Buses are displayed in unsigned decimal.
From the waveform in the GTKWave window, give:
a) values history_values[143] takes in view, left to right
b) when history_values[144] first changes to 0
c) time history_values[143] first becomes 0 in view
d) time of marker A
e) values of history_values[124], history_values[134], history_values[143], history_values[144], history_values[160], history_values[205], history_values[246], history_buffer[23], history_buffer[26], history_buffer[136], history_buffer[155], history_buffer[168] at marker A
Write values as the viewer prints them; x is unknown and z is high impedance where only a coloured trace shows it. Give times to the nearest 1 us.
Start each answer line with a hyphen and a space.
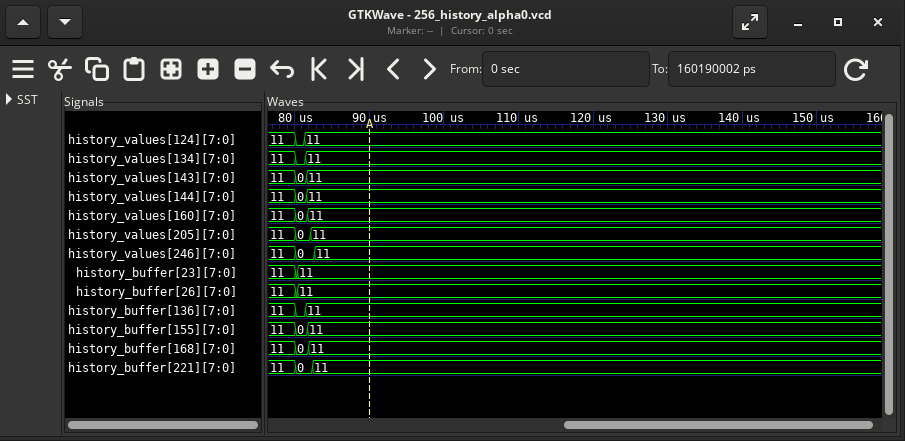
- 11, 0, 11
- 80 us
- 80 us
- 90 us
- history_values[124]=11, history_values[134]=11, history_values[143]=11, history_values[144]=11, history_values[160]=11, history_values[205]=11, history_values[246]=11, history_buffer[23]=11, history_buffer[26]=11, history_buffer[136]=11, history_buffer[155]=11, history_buffer[168]=11
